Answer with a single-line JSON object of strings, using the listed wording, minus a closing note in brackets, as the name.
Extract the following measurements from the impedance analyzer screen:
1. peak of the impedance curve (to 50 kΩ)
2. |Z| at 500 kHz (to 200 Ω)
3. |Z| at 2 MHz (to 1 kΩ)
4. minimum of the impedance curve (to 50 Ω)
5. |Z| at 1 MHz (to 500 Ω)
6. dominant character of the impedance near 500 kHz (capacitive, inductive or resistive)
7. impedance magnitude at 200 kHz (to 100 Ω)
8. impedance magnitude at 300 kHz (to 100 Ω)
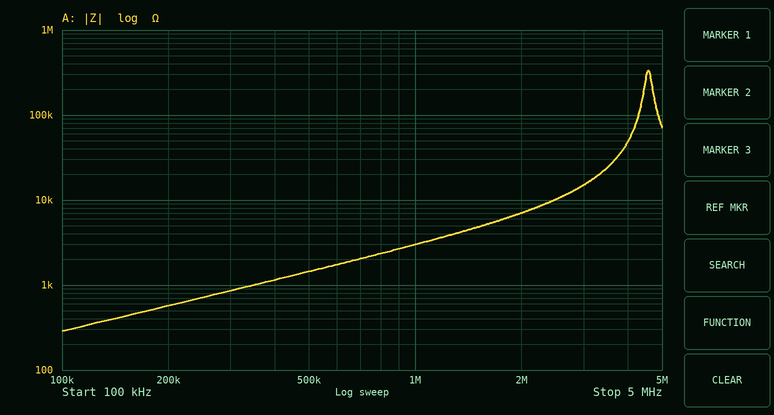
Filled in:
{"peak of the impedance curve": "350 kΩ", "|Z| at 500 kHz": "1.4 kΩ", "|Z| at 2 MHz": "7 kΩ", "minimum of the impedance curve": "300 Ω", "|Z| at 1 MHz": "3.0 kΩ", "dominant character of the impedance near 500 kHz": "inductive", "impedance magnitude at 200 kHz": "600 Ω", "impedance magnitude at 300 kHz": "900 Ω"}
